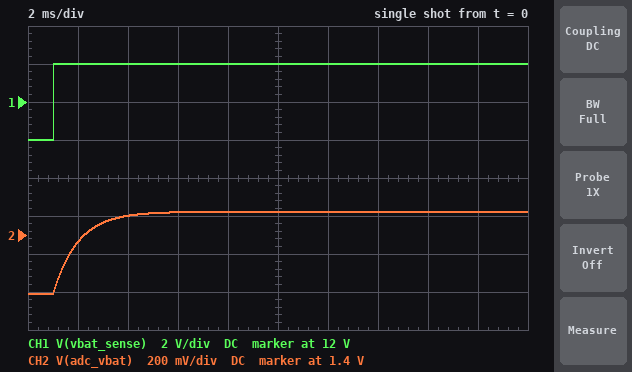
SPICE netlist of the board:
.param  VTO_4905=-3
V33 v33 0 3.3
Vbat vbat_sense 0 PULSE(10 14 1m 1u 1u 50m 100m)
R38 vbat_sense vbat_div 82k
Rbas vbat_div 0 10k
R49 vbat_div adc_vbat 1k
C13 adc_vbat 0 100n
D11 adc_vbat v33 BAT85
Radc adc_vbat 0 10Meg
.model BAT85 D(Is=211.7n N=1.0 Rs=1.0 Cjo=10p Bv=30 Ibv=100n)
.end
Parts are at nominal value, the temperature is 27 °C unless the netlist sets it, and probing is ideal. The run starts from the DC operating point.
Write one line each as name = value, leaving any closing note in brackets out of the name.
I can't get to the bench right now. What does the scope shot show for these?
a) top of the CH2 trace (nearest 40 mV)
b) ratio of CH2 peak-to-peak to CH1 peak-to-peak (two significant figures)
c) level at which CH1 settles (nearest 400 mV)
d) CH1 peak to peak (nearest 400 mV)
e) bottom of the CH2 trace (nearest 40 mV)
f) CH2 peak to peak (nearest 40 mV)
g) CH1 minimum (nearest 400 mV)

top of the CH2 trace = 1.52 V
ratio of CH2 peak-to-peak to CH1 peak-to-peak = 0.11
level at which CH1 settles = 14.0 V
CH1 peak to peak = 4.0 V
bottom of the CH2 trace = 1.08 V
CH2 peak to peak = 440 mV
CH1 minimum = 10.0 V
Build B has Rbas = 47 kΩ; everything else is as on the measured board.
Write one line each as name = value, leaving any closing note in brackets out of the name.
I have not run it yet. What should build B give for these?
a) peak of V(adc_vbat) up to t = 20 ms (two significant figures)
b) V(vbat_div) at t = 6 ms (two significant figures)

peak of V(adc_vbat) up to t = 20 ms = 3.4 V
V(vbat_div) at t = 6 ms = 3.5 V
